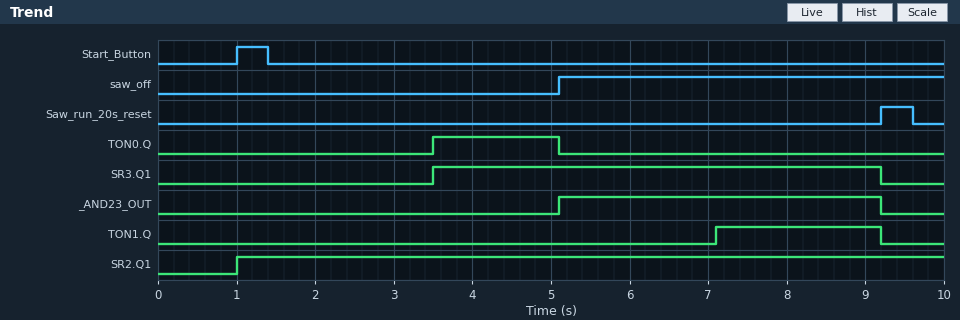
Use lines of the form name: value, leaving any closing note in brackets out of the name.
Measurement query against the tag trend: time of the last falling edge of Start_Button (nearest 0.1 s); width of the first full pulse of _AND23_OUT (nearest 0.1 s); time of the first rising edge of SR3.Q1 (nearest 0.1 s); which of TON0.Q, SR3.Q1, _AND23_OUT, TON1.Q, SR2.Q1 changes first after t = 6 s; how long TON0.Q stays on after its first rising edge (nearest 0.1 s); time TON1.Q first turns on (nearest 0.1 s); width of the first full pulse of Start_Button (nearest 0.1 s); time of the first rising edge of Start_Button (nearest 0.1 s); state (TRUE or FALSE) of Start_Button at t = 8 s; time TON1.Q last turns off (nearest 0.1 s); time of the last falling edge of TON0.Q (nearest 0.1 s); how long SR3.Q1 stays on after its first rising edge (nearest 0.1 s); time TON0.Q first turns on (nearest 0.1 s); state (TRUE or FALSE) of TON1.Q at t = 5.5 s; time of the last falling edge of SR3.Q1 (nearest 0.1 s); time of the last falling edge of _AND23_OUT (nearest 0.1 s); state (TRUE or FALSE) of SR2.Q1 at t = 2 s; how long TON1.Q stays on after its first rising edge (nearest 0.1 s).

time of the last falling edge of Start_Button: 1.4 s
width of the first full pulse of _AND23_OUT: 4.1 s
time of the first rising edge of SR3.Q1: 3.5 s
which of TON0.Q, SR3.Q1, _AND23_OUT, TON1.Q, SR2.Q1 changes first after t = 6 s: TON1.Q
how long TON0.Q stays on after its first rising edge: 1.6 s
time TON1.Q first turns on: 7.1 s
width of the first full pulse of Start_Button: 0.4 s
time of the first rising edge of Start_Button: 1.0 s
state (TRUE or FALSE) of Start_Button at t = 8 s: FALSE
time TON1.Q last turns off: 9.2 s
time of the last falling edge of TON0.Q: 5.1 s
how long SR3.Q1 stays on after its first rising edge: 5.7 s
time TON0.Q first turns on: 3.5 s
state (TRUE or FALSE) of TON1.Q at t = 5.5 s: FALSE
time of the last falling edge of SR3.Q1: 9.2 s
time of the last falling edge of _AND23_OUT: 9.2 s
state (TRUE or FALSE) of SR2.Q1 at t = 2 s: TRUE
how long TON1.Q stays on after its first rising edge: 2.1 s
